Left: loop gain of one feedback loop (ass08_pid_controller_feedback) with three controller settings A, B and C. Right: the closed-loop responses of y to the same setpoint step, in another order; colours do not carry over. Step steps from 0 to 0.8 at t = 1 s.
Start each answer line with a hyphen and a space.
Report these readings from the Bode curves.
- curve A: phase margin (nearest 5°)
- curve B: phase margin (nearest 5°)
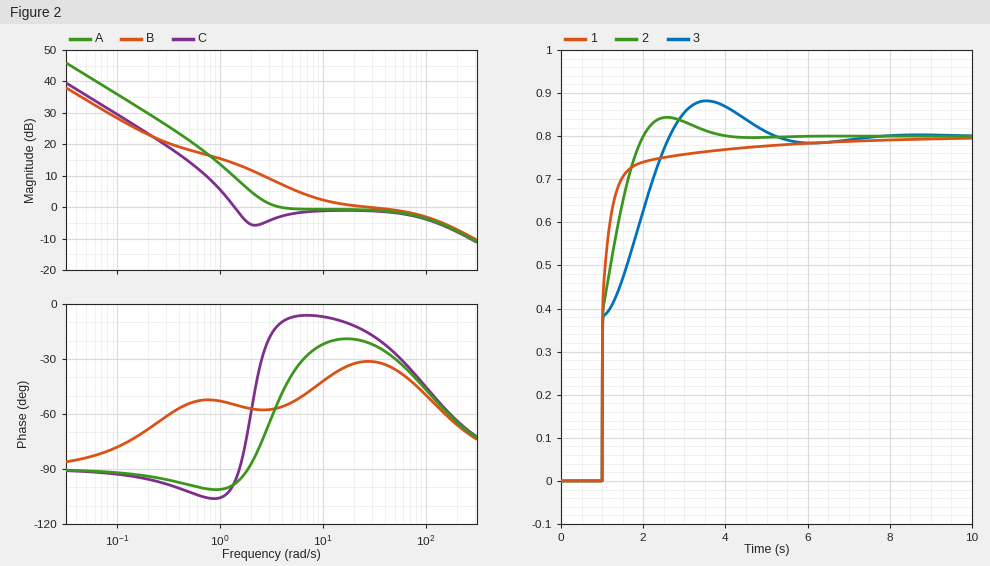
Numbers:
- 130°
- 150°
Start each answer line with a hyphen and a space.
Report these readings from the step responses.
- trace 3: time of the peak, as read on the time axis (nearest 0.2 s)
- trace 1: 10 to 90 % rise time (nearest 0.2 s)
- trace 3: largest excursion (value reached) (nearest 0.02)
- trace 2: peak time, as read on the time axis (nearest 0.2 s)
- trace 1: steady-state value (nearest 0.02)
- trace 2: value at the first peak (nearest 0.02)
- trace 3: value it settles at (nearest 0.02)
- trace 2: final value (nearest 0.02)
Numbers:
- 3.6 s
- 0.6 s
- 0.88
- 2.6 s
- 0.80
- 0.84
- 0.80
- 0.80
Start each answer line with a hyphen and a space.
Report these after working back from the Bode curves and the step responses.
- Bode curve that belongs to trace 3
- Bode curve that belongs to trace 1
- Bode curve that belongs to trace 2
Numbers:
- C
- B
- A
